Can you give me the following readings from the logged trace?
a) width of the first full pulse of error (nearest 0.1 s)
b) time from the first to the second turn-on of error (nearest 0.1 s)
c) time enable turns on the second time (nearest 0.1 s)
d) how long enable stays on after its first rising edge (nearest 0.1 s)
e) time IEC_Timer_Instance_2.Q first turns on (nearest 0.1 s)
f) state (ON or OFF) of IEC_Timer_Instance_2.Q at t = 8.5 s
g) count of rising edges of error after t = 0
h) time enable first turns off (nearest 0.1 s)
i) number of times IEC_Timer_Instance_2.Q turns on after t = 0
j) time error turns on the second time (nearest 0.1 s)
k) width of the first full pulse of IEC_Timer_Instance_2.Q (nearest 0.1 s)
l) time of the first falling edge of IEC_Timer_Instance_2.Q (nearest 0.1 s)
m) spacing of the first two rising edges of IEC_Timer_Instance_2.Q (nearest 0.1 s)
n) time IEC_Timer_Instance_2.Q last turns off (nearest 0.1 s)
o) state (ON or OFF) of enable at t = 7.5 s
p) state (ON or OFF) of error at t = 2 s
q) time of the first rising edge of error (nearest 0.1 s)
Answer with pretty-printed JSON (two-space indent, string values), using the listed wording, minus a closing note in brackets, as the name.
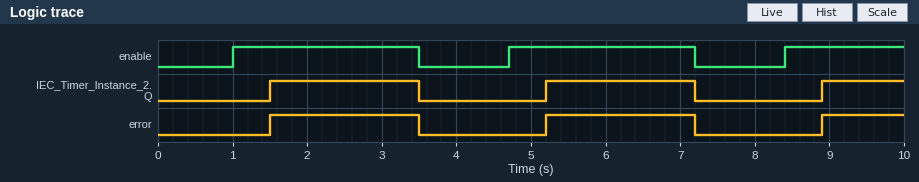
{
  "width of the first full pulse of error": "2.0 s",
  "time from the first to the second turn-on of error": "3.7 s",
  "time enable turns on the second time": "4.7 s",
  "how long enable stays on after its first rising edge": "2.5 s",
  "time IEC_Timer_Instance_2.Q first turns on": "1.5 s",
  "state (ON or OFF) of IEC_Timer_Instance_2.Q at t = 8.5 s": "OFF",
  "count of rising edges of error after t = 0": "3",
  "time enable first turns off": "3.5 s",
  "number of times IEC_Timer_Instance_2.Q turns on after t = 0": "3",
  "time error turns on the second time": "5.2 s",
  "width of the first full pulse of IEC_Timer_Instance_2.Q": "2.0 s",
  "time of the first falling edge of IEC_Timer_Instance_2.Q": "3.5 s",
  "spacing of the first two rising edges of IEC_Timer_Instance_2.Q": "3.7 s",
  "time IEC_Timer_Instance_2.Q last turns off": "7.2 s",
  "state (ON or OFF) of enable at t = 7.5 s": "OFF",
  "state (ON or OFF) of error at t = 2 s": "ON",
  "time of the first rising edge of error": "1.5 s"
}
